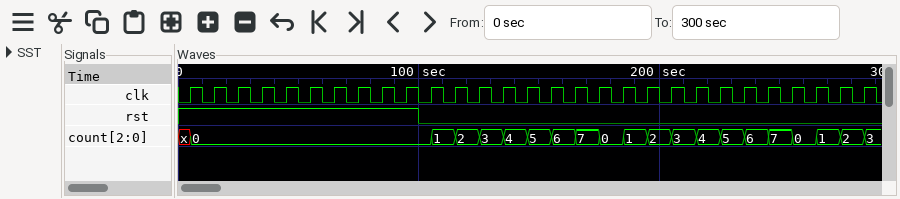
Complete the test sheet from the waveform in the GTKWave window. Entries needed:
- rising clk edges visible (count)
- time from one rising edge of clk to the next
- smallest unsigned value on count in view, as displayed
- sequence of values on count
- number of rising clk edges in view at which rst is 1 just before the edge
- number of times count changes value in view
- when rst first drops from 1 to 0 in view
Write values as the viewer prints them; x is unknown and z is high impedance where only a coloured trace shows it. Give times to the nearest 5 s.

29
10 s
0
x, 0, 1, 2, 3, 4, 5, 6, 7, 0, 1, 2, 3, 4, 5, 6, 7, 0, 1, 2, 3
10
20
100 s
